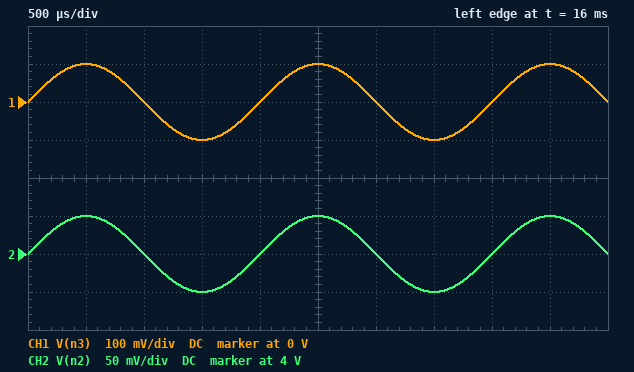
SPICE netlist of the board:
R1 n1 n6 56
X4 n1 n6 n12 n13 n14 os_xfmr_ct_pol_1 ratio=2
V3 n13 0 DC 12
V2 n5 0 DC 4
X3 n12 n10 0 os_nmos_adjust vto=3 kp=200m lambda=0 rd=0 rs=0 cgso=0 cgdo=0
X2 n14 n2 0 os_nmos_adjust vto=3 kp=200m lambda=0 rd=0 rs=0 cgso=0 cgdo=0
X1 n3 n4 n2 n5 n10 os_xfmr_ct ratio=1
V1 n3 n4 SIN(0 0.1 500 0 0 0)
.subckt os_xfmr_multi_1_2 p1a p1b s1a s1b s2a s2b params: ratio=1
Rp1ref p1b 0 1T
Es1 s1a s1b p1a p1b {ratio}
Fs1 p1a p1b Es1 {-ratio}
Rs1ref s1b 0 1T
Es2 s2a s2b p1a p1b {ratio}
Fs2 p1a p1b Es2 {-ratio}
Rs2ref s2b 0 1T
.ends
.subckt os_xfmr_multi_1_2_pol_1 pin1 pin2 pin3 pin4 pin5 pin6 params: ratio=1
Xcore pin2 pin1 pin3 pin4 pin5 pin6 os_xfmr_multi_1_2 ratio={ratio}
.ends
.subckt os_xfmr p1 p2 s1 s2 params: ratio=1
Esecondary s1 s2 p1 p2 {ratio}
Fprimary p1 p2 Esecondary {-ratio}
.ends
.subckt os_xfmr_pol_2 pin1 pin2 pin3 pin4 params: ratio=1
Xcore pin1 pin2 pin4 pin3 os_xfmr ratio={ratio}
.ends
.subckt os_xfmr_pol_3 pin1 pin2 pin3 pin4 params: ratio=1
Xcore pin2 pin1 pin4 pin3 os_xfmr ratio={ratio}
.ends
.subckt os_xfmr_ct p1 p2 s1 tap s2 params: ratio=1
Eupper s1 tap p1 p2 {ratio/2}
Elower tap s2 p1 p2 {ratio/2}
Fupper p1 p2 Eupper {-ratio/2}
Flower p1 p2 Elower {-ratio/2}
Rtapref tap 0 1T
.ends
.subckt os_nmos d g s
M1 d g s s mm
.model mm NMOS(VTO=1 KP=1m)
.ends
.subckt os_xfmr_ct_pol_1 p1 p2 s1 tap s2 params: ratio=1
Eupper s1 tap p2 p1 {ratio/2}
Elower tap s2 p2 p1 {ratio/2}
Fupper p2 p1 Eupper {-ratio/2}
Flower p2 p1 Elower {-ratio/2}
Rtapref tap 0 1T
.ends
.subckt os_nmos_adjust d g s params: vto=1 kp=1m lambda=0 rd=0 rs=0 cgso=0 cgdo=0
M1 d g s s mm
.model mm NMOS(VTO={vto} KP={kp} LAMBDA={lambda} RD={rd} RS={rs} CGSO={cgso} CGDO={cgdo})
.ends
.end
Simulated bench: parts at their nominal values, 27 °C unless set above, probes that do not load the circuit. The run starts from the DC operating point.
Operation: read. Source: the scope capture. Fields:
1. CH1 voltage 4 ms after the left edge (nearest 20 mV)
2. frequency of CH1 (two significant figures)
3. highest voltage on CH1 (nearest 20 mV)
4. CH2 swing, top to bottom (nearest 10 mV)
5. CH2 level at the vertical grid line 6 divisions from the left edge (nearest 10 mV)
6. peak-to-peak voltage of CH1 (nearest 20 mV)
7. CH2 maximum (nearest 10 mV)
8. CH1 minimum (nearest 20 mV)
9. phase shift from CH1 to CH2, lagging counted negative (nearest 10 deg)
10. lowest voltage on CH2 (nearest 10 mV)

0 V
500 Hz
100 mV
100 mV
4.00 V
200 mV
4.05 V
-100 mV
0 deg
3.95 V
